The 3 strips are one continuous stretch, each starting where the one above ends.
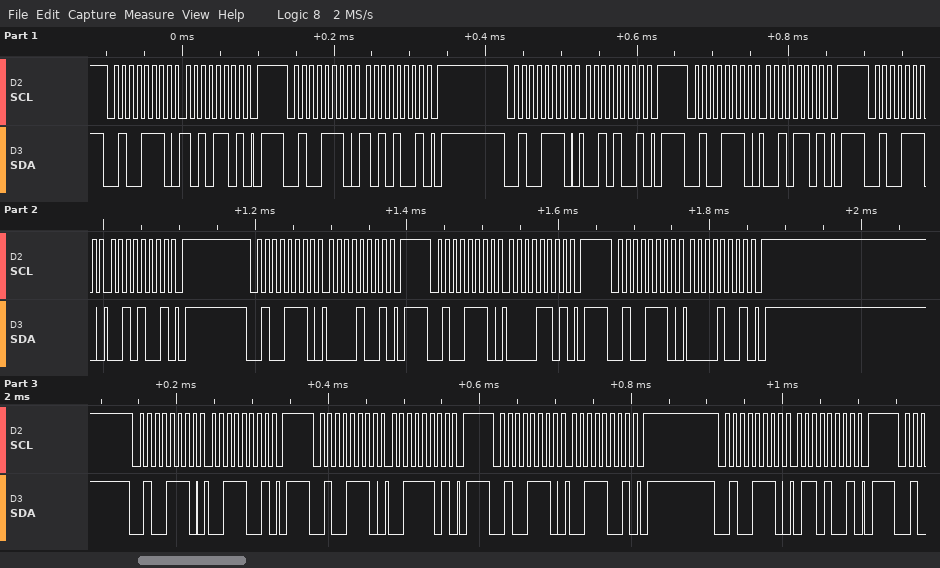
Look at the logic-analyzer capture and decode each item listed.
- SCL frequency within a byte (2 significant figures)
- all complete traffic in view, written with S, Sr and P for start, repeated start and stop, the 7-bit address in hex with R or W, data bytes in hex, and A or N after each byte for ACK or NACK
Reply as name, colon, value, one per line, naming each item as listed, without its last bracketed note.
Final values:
SCL frequency within a byte: 100 kHz
all complete traffic in view, written with S, Sr and P for start, repeated start and stop, the 7-bit address in hex with R or W, data bytes in hex, and A or N after each byte for ACK or NACK: S 27W A AD A P S 27W A A9 A P S 27W A 29 A P S 27W A 2D A P S 27W A 29 A P S 27W A 09 A P S 27W A 0D A P S 27W A 09 A P S 27W A 39 A P S 27W A 3D A P S 27W A 39 A P S 27W A 69 A P
